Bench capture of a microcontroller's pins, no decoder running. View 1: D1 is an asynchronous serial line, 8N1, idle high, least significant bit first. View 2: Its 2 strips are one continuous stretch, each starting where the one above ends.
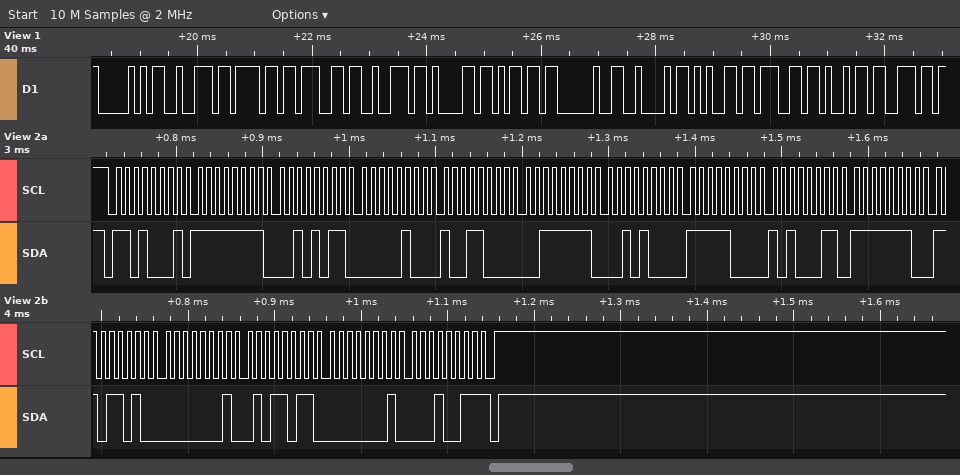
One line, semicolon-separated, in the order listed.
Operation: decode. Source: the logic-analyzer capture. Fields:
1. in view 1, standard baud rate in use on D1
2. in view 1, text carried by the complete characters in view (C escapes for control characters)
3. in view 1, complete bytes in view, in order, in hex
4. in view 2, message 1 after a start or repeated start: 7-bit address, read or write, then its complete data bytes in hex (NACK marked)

9600 baud; "Program Begin"; 50 72 6F 67 72 61 6D 20 42 65 67 69 6E; 0x68 read: FF 2B 04 98 3F 28 F8 A3 FE DA 01 5B 01 13 NACK
